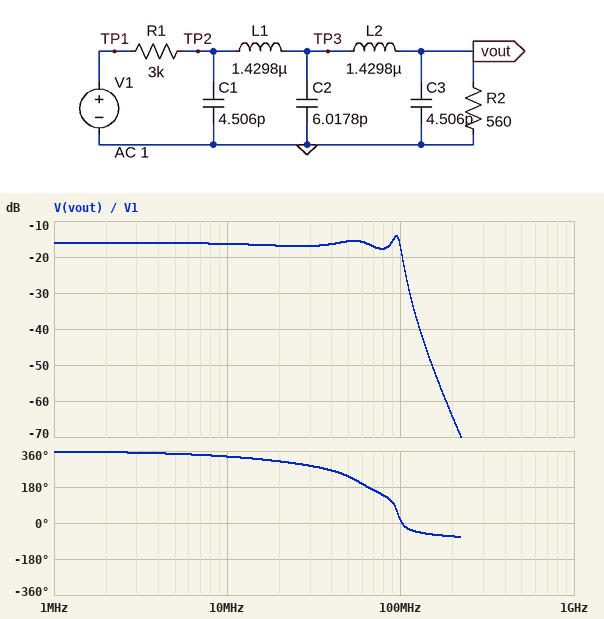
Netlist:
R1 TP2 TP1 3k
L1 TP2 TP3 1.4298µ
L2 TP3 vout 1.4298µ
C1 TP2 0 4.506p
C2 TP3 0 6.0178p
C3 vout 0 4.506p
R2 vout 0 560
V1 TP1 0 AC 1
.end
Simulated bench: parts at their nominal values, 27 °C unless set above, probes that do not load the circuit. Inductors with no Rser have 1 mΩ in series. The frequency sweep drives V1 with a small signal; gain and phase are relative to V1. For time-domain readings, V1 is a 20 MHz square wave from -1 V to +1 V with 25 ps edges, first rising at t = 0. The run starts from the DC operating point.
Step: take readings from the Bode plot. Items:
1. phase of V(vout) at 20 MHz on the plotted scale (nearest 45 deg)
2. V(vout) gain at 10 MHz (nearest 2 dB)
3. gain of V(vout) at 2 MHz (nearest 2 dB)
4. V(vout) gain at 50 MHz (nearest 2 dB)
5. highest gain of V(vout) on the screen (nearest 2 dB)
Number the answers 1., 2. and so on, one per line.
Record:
1. 315 deg
2. -16 dB
3. -16 dB
4. -16 dB
5. -14 dB
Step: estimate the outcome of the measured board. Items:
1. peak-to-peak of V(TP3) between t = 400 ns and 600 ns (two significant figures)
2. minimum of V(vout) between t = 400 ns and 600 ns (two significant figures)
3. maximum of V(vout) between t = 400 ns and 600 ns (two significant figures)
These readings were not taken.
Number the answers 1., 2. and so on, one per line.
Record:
1. 450 mV
2. -210 mV
3. 210 mV
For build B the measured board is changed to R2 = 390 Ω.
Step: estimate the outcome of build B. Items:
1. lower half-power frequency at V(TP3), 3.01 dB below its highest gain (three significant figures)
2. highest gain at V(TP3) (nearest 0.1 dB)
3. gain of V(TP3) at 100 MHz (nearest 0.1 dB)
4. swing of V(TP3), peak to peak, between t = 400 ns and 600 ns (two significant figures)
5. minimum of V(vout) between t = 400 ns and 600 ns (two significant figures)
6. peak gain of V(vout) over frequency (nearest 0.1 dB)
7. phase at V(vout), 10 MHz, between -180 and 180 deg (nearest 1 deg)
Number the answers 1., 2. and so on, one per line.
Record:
1. 87.4 MHz
2. -7.5 dB
3. -11.4 dB
4. 490 mV
5. -180 mV
6. -15.4 dB
7. -22 deg
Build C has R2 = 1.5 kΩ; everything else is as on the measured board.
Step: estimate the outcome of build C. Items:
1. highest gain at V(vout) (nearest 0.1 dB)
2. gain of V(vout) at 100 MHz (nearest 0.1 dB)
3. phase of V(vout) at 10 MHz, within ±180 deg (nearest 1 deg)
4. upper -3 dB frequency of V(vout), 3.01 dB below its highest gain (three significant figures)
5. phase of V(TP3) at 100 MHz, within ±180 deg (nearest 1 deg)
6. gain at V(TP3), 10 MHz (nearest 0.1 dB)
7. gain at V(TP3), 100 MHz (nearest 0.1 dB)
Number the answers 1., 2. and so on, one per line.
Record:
1. -9.4 dB
2. -10.8 dB
3. -46 deg
4. 101 MHz
5. 159 deg
6. -12.2 dB
7. -6.4 dB
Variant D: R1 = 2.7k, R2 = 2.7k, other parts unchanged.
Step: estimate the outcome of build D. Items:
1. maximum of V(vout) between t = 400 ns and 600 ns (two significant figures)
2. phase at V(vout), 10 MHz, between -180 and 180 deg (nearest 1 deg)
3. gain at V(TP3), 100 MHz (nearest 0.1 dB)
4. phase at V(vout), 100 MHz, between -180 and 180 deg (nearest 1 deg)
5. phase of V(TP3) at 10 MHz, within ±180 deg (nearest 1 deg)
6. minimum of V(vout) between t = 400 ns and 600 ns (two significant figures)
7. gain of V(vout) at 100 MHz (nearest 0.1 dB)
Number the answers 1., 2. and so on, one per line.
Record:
1. 370 mV
2. -54 deg
3. -3.4 dB
4. -6 deg
5. -52 deg
6. -370 mV
7. -7.3 dB
